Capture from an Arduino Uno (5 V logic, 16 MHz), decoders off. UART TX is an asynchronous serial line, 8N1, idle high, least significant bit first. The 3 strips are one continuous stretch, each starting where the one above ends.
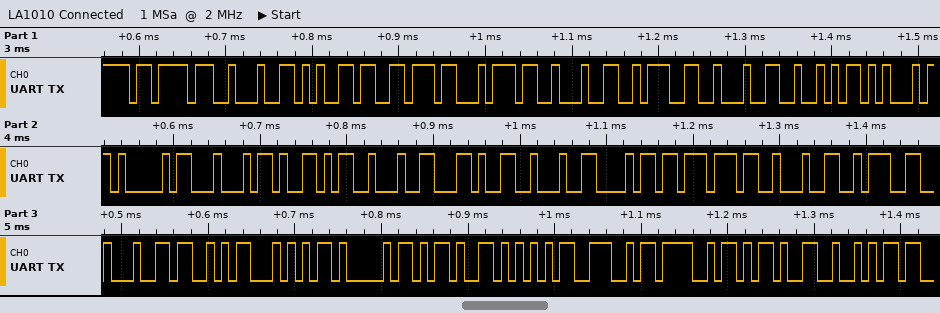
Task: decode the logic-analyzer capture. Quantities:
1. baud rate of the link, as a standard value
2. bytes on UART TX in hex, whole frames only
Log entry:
115200 baud
7B 22 65 76 74 22 3A 22 52 45 41 44 59 22 2C 22 68 77 22 3A 22 53 54 41 2D 55 4E 4F 2D 52
